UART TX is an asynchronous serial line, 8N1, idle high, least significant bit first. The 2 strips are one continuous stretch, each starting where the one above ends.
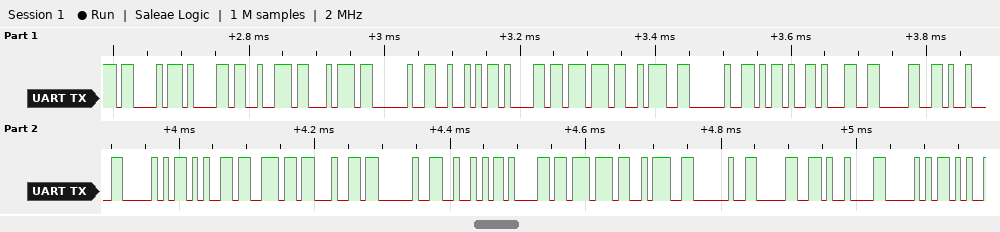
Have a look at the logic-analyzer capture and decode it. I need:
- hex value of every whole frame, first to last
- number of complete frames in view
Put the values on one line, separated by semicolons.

43 61 72 74 20 52 61 77 3A 20 2D 31 30 09 50 65 6E 64 20 52 61 77 3A 20 30 09 50; 27
